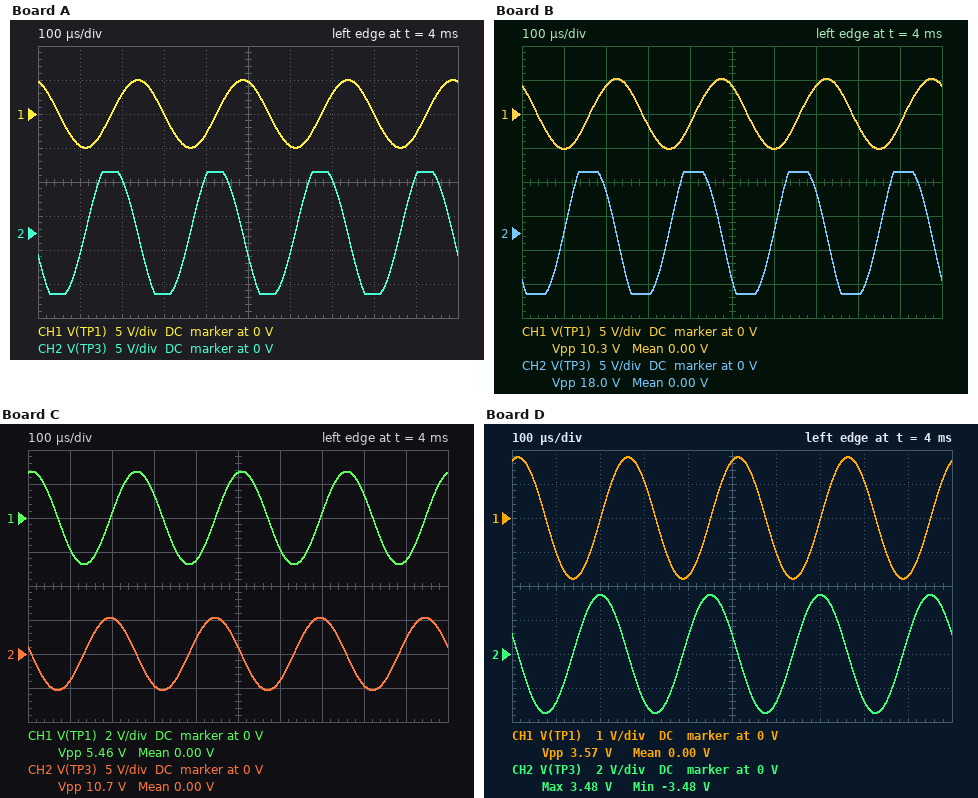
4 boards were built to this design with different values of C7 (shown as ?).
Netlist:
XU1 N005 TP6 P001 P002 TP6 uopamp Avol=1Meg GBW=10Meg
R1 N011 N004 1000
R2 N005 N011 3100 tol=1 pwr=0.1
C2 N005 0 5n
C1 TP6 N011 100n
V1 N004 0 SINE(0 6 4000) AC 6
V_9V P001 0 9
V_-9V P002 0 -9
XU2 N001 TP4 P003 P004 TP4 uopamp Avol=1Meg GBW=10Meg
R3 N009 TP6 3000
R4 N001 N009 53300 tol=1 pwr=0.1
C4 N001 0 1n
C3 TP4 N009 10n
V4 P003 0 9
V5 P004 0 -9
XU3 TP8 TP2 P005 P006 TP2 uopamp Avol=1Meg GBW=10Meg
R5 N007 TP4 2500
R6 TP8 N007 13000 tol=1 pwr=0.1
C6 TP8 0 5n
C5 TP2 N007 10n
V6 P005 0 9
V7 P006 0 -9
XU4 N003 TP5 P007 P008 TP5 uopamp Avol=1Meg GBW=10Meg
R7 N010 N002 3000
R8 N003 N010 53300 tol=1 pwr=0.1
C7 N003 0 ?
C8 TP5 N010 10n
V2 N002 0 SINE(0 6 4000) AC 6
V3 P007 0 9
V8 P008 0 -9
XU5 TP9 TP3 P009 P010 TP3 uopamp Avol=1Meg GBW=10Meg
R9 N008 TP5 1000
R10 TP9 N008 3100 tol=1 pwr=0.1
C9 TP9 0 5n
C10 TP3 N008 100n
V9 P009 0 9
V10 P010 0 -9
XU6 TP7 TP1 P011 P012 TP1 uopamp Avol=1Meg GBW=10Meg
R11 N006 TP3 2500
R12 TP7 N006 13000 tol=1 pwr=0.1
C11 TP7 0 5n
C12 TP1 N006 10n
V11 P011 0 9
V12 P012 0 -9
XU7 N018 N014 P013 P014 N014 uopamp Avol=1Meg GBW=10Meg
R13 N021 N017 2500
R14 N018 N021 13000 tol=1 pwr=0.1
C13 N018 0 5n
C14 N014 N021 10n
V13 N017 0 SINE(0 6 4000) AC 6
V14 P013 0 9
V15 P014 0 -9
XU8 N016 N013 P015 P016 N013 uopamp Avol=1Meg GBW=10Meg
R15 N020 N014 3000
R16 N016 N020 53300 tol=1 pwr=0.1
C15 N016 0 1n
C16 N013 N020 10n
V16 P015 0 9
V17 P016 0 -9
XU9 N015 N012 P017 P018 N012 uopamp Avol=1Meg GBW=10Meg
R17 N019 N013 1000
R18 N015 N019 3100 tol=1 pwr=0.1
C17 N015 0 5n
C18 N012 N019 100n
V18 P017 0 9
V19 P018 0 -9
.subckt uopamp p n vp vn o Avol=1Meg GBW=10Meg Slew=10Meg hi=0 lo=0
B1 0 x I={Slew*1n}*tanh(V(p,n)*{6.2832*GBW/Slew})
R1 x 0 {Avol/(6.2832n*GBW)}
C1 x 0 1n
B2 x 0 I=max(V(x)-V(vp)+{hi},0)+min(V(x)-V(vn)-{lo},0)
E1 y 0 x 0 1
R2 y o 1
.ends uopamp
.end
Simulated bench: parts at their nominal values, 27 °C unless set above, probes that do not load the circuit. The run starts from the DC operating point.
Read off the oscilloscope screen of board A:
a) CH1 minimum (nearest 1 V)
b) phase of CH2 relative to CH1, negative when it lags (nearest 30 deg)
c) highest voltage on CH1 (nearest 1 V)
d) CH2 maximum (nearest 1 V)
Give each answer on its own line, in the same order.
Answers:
-5 V
90 deg
5 V
9 V
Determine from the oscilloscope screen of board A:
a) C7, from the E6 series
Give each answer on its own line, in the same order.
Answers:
680 pF
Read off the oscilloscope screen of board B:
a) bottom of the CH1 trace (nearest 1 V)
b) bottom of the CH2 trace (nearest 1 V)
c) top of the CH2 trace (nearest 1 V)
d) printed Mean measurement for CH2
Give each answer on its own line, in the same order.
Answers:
-5 V
-9 V
9 V
0.00 V
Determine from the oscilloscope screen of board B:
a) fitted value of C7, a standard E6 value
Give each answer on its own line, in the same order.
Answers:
470 pF
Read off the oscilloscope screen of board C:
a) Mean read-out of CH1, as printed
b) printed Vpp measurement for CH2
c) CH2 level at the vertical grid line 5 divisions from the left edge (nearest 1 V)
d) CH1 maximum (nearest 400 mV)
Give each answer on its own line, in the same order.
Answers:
0.00 V
10.7 V
1 V
2.8 V
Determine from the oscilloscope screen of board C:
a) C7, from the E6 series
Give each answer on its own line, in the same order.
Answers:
1.5 nF
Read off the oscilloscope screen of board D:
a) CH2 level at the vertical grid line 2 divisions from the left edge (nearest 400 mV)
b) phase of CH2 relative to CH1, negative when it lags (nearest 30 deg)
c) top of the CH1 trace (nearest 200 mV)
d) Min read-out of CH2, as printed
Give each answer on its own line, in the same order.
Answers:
3.6 V
90 deg
1.8 V
-3.48 V
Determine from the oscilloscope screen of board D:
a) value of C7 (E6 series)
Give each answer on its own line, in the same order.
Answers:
2.2 nF
